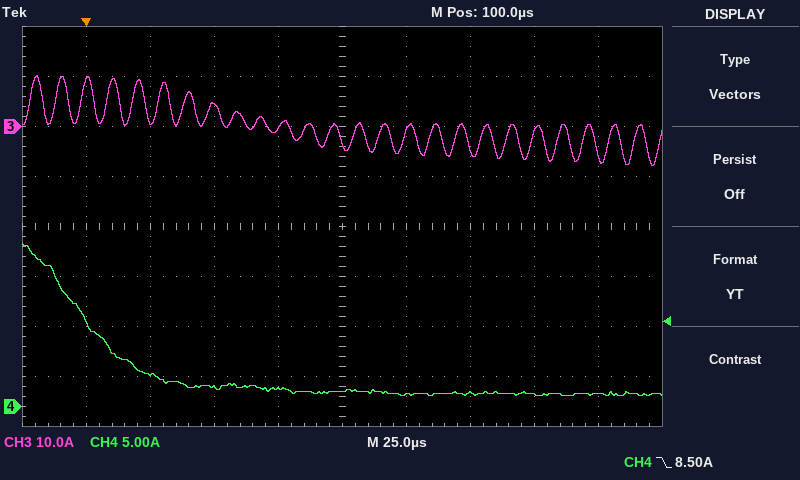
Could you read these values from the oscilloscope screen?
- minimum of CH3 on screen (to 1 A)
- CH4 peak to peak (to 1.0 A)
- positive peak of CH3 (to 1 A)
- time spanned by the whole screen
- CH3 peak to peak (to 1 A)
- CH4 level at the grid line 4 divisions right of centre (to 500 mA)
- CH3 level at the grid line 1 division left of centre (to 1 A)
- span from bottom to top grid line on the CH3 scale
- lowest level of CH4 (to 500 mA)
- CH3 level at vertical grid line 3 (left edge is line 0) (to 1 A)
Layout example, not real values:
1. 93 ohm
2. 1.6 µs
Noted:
1. -8 A
2. 15.0 A
3. 10 A
4. 250 µs
5. 18 A
6. 1.5 A
7. 0 A
8. 80 A
9. 1.0 A
10. 4 A
